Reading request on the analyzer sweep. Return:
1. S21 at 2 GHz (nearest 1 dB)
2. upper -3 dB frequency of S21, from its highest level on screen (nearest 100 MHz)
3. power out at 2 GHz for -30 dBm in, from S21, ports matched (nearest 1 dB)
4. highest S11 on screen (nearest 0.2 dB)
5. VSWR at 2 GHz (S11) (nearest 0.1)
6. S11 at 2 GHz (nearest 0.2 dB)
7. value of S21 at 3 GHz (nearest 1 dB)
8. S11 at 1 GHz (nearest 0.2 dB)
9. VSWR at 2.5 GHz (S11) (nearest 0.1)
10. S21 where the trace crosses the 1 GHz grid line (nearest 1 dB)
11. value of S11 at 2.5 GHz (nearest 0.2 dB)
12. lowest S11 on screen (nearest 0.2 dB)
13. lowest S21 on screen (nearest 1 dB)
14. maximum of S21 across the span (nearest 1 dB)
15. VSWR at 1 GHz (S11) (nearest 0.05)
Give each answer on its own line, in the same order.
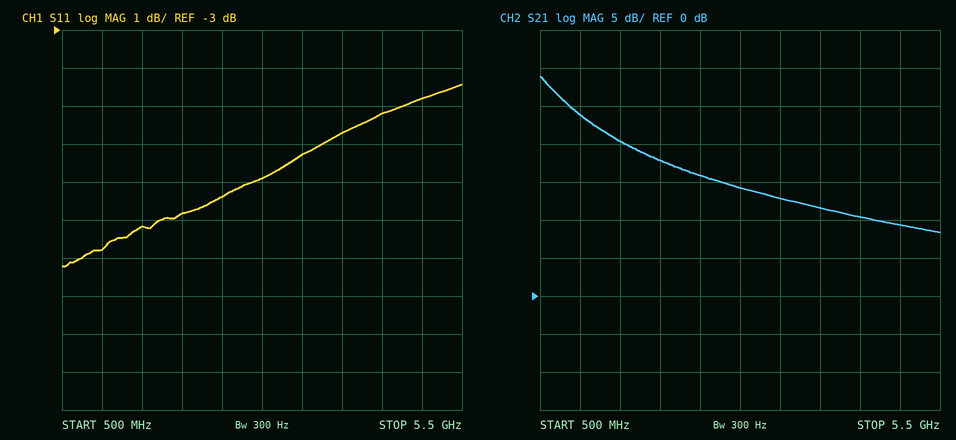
18 dB
800 MHz
-12 dBm
-4.4 dB
2.4
-7.8 dB
14 dB
-8.8 dB
2.5
24 dB
-7.4 dB
-9.2 dB
8 dB
29 dB
2.15
